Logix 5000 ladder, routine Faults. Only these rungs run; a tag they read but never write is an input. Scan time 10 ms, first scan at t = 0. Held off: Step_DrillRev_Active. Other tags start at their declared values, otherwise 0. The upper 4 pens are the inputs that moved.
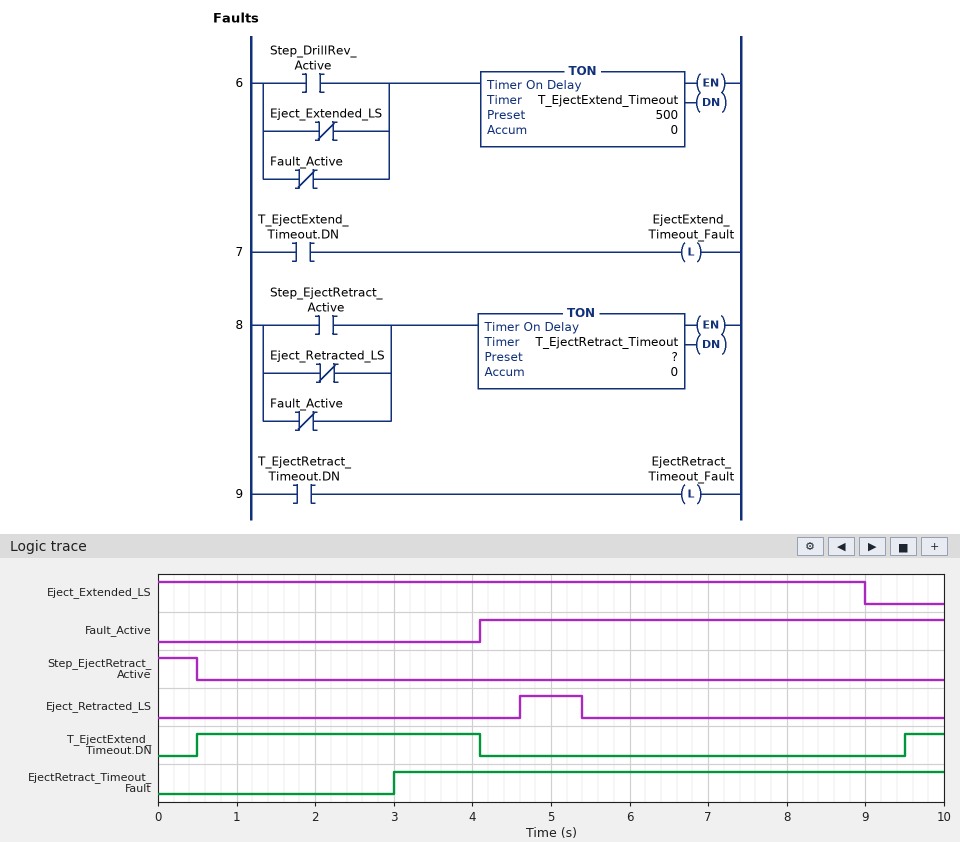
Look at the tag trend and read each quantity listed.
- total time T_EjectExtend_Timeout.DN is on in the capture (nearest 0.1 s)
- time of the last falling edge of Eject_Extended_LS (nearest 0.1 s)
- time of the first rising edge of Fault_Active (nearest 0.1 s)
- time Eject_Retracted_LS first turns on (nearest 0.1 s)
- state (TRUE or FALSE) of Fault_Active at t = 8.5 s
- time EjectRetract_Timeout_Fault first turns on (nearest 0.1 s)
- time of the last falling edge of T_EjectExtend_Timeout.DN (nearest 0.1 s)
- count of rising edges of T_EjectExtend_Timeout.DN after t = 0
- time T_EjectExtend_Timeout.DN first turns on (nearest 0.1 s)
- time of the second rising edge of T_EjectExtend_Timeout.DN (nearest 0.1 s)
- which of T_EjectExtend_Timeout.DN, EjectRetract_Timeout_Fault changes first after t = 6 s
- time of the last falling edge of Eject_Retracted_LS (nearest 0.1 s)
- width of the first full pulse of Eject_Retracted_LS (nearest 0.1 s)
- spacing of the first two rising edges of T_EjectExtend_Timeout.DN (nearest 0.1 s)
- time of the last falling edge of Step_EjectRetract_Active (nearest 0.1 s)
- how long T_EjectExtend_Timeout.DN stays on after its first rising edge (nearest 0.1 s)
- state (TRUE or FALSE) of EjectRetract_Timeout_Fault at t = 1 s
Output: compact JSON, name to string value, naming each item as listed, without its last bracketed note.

{"total time T_EjectExtend_Timeout.DN is on in the capture": "4.1 s", "time of the last falling edge of Eject_Extended_LS": "9.0 s", "time of the first rising edge of Fault_Active": "4.1 s", "time Eject_Retracted_LS first turns on": "4.6 s", "state (TRUE or FALSE) of Fault_Active at t = 8.5 s": "TRUE", "time EjectRetract_Timeout_Fault first turns on": "3.0 s", "time of the last falling edge of T_EjectExtend_Timeout.DN": "4.1 s", "count of rising edges of T_EjectExtend_Timeout.DN after t = 0": "2", "time T_EjectExtend_Timeout.DN first turns on": "0.5 s", "time of the second rising edge of T_EjectExtend_Timeout.DN": "9.5 s", "which of T_EjectExtend_Timeout.DN, EjectRetract_Timeout_Fault changes first after t = 6 s": "T_EjectExtend_Timeout.DN", "time of the last falling edge of Eject_Retracted_LS": "5.4 s", "width of the first full pulse of Eject_Retracted_LS": "0.8 s", "spacing of the first two rising edges of T_EjectExtend_Timeout.DN": "9.0 s", "time of the last falling edge of Step_EjectRetract_Active": "0.5 s", "how long T_EjectExtend_Timeout.DN stays on after its first rising edge": "3.6 s", "state (TRUE or FALSE) of EjectRetract_Timeout_Fault at t = 1 s": "FALSE"}
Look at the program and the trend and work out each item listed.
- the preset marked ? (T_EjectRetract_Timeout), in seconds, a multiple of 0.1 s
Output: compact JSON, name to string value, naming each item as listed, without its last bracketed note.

{"the preset marked ? (T_EjectRetract_Timeout), in seconds, a multiple of 0.1 s": "3.0 s"}
